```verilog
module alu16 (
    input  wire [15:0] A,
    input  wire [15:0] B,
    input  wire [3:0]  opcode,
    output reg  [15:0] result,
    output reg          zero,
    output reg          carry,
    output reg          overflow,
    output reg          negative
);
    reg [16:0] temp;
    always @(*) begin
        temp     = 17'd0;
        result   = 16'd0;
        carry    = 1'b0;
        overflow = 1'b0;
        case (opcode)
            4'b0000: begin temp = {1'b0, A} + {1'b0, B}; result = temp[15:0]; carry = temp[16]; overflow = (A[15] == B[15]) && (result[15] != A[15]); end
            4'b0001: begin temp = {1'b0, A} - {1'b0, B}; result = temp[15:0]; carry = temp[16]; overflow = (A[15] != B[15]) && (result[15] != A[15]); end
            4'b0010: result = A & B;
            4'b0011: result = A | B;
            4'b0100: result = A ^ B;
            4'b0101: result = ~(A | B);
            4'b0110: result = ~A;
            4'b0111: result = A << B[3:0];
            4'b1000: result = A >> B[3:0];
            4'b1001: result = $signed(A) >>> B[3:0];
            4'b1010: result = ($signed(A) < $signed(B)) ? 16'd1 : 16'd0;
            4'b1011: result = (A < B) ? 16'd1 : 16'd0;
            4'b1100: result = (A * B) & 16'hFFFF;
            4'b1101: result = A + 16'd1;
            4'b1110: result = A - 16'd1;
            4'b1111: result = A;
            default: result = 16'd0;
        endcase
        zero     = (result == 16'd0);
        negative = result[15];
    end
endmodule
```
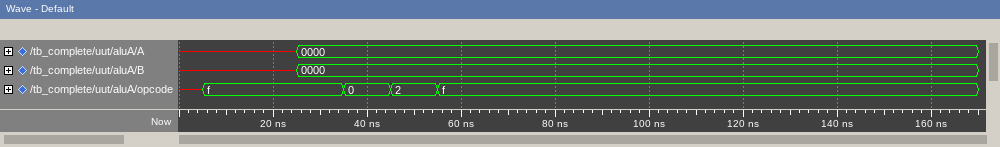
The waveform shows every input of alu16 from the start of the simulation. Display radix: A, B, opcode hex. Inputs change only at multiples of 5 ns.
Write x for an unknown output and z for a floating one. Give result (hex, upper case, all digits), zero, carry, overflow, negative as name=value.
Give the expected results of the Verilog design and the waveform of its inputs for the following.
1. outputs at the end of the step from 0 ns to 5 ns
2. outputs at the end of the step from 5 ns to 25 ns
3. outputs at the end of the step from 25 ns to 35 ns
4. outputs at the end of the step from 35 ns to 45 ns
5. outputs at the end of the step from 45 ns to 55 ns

result=x, zero=x, carry=x, overflow=x, negative=x
result=x, zero=x, carry=0, overflow=0, negative=x
result=0000, zero=1, carry=0, overflow=0, negative=0
result=0000, zero=1, carry=0, overflow=0, negative=0
result=0000, zero=1, carry=0, overflow=0, negative=0
